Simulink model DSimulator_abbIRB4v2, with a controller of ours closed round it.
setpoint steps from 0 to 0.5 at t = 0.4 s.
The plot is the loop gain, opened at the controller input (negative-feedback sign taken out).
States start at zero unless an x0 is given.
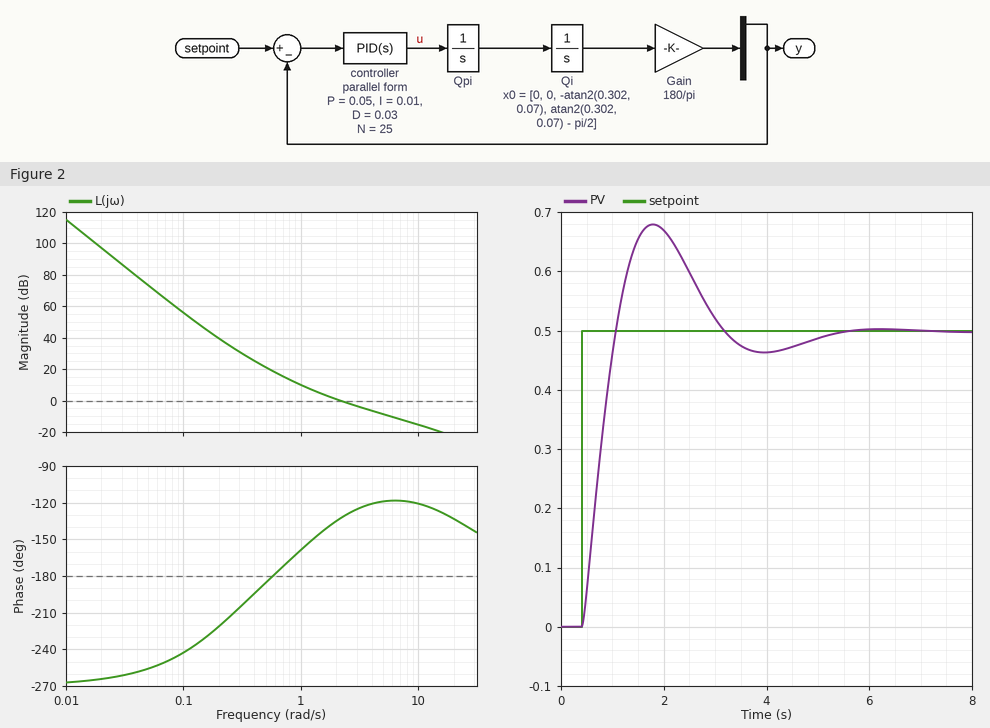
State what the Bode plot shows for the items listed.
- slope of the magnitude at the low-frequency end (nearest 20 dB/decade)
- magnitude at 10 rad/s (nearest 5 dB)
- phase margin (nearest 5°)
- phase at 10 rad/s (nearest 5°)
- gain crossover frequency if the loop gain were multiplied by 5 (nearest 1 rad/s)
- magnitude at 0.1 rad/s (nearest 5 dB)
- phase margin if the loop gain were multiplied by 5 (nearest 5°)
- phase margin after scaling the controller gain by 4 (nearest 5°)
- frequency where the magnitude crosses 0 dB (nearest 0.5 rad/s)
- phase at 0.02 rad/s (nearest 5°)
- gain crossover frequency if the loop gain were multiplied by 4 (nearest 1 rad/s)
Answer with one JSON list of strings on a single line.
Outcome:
["-60 dB/decade", "-15 dB", "45°", "-120°", "9 rad/s", "55 dB", "60°", "60°", "2.0 rad/s", "-265°", "7 rad/s"]
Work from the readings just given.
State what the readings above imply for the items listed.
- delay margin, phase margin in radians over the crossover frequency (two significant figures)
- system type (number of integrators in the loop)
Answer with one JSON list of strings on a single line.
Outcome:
["0.39 s", "3"]
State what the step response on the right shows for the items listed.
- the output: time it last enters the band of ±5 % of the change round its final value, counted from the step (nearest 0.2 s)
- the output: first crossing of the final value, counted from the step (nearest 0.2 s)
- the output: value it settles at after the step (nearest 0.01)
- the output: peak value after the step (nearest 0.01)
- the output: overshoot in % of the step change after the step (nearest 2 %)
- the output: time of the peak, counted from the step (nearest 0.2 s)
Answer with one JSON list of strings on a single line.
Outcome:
["4.2 s", "0.6 s", "0.50", "0.68", "36 %", "1.4 s"]
